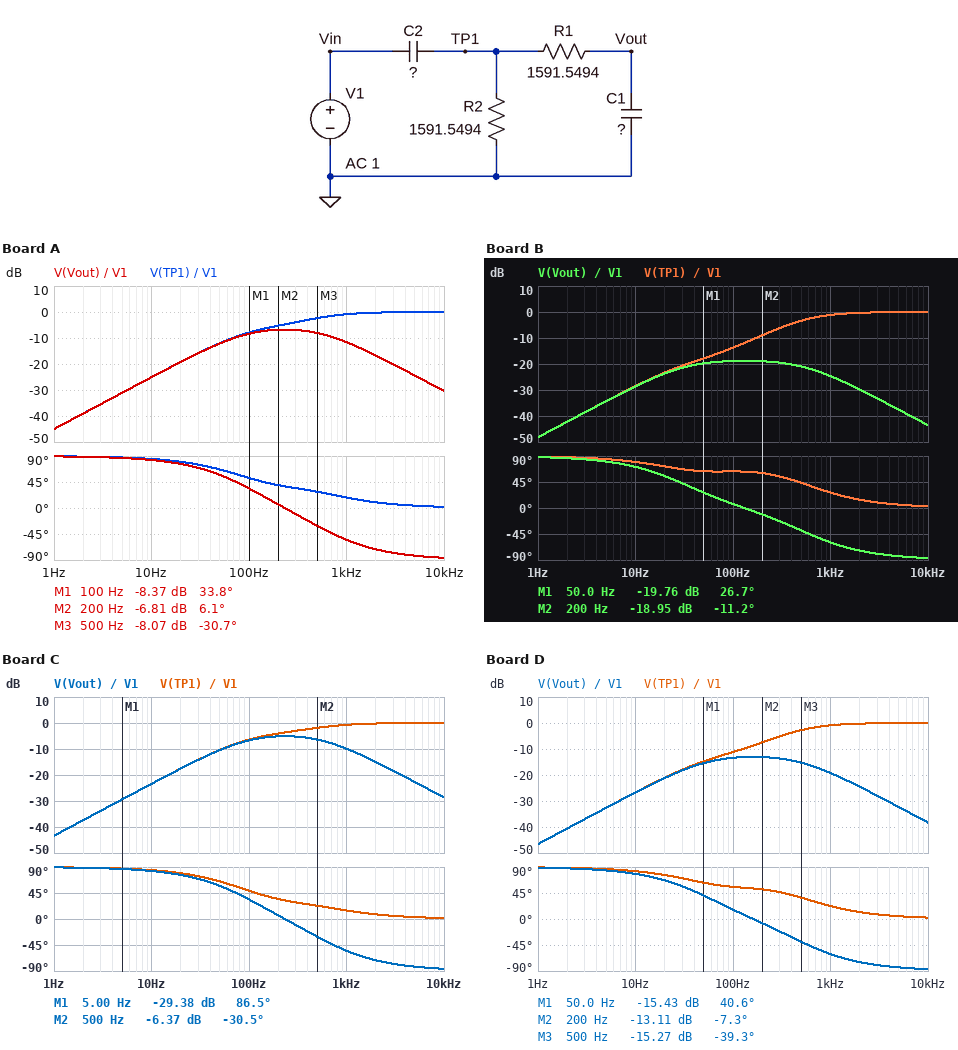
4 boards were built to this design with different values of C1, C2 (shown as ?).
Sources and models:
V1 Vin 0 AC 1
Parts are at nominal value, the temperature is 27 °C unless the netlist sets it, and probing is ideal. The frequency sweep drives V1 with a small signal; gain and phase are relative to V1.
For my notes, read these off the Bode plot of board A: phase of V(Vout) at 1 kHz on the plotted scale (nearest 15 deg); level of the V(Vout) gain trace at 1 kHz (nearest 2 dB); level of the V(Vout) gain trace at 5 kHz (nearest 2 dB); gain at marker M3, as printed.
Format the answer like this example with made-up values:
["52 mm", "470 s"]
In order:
["-60 deg", "-12 dB", "-24 dB", "-8.07 dB"]
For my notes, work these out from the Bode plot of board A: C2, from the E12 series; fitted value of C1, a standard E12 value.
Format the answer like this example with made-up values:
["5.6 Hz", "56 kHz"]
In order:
["560 nF", "330 nF"]
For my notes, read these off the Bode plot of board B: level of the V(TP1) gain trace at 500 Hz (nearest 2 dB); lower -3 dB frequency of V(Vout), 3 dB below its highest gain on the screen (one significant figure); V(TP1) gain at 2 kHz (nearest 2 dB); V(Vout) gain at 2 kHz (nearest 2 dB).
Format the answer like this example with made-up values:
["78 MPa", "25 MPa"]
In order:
["-4 dB", "30 Hz", "0 dB", "-30 dB"]
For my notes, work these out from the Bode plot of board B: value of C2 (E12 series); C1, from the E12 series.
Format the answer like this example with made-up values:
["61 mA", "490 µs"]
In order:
["390 nF", "1.5 µF"]
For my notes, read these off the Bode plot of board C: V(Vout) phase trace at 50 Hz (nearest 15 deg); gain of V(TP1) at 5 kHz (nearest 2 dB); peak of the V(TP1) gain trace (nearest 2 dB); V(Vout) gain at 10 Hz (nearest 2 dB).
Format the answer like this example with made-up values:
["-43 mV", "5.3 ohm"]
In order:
["60 deg", "0 dB", "0 dB", "-24 dB"]
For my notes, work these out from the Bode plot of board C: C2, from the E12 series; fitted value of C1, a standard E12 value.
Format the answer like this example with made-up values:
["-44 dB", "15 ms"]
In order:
["680 nF", "270 nF"]
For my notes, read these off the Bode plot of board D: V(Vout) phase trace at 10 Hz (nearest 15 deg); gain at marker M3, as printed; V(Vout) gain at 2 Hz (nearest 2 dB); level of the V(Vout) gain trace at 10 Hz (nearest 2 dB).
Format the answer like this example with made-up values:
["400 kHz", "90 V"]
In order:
["75 deg", "-15.27 dB", "-40 dB", "-26 dB"]
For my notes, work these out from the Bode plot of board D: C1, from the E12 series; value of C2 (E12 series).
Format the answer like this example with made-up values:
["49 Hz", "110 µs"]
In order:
["820 nF", "470 nF"]
